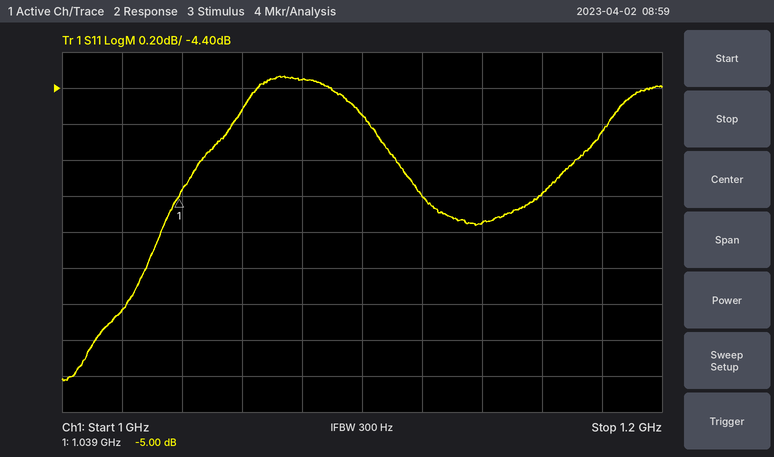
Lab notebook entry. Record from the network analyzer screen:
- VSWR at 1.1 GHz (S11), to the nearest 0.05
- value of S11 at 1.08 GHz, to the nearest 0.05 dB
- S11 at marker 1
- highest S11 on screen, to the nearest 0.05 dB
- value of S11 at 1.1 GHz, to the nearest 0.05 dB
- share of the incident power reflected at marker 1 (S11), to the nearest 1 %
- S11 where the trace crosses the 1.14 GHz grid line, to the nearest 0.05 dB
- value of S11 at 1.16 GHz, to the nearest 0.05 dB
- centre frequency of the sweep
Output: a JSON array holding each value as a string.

["3.90", "-4.35 dB", "-5.00 dB", "-4.35 dB", "-4.55 dB", "32 %", "-5.15 dB", "-5.00 dB", "1.1 GHz"]
